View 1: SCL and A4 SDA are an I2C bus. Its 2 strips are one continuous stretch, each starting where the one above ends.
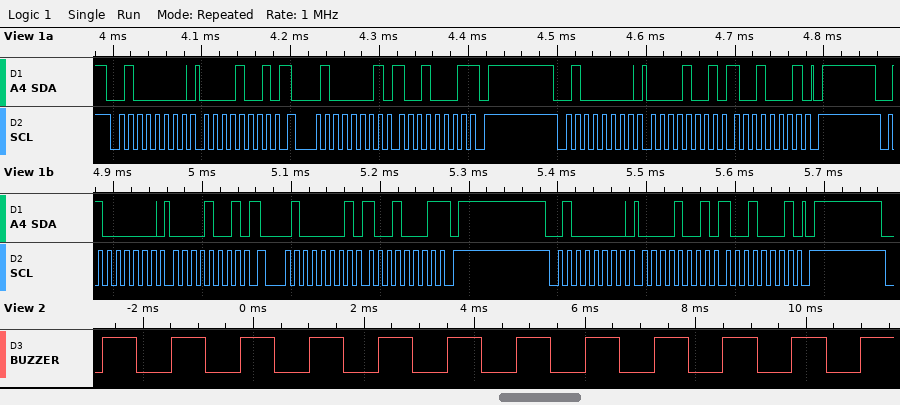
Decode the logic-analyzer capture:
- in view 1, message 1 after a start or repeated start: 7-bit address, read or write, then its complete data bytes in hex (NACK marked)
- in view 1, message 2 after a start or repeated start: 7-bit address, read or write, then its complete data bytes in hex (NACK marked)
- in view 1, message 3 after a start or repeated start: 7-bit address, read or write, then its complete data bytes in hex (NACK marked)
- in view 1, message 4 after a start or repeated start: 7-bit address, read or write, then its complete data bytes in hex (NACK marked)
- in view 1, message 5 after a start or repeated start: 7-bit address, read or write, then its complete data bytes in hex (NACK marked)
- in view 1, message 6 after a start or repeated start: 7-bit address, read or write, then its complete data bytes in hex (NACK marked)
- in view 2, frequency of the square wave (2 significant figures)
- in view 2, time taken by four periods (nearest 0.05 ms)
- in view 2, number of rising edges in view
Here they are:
0x20 write: 09
0x20 read: 91 NACK
0x20 write: 09 91
0x20 write: 09
0x20 read: 91 NACK
0x20 write: 09 91
800 Hz
5.00 ms
12
